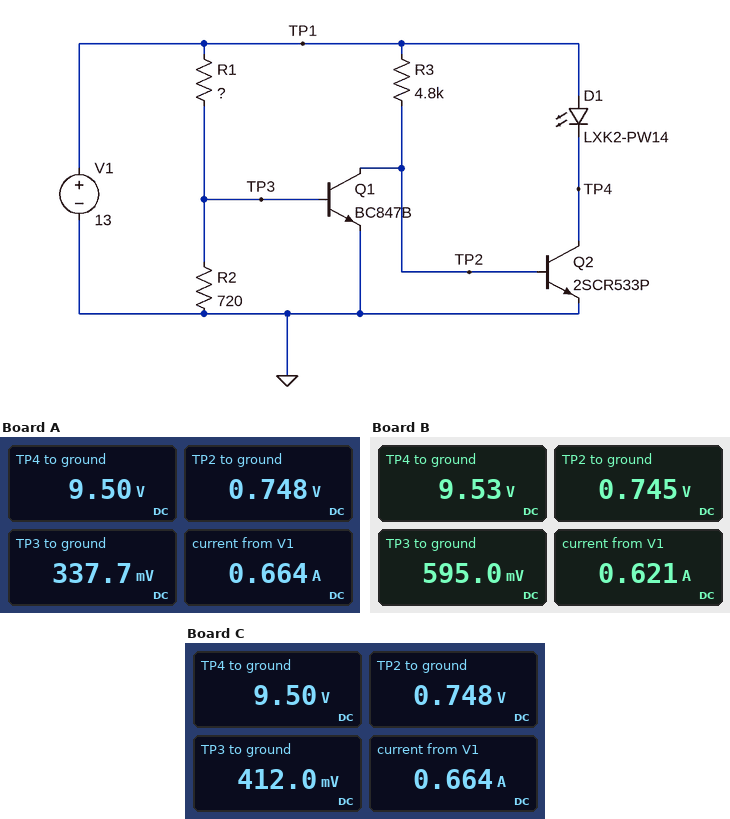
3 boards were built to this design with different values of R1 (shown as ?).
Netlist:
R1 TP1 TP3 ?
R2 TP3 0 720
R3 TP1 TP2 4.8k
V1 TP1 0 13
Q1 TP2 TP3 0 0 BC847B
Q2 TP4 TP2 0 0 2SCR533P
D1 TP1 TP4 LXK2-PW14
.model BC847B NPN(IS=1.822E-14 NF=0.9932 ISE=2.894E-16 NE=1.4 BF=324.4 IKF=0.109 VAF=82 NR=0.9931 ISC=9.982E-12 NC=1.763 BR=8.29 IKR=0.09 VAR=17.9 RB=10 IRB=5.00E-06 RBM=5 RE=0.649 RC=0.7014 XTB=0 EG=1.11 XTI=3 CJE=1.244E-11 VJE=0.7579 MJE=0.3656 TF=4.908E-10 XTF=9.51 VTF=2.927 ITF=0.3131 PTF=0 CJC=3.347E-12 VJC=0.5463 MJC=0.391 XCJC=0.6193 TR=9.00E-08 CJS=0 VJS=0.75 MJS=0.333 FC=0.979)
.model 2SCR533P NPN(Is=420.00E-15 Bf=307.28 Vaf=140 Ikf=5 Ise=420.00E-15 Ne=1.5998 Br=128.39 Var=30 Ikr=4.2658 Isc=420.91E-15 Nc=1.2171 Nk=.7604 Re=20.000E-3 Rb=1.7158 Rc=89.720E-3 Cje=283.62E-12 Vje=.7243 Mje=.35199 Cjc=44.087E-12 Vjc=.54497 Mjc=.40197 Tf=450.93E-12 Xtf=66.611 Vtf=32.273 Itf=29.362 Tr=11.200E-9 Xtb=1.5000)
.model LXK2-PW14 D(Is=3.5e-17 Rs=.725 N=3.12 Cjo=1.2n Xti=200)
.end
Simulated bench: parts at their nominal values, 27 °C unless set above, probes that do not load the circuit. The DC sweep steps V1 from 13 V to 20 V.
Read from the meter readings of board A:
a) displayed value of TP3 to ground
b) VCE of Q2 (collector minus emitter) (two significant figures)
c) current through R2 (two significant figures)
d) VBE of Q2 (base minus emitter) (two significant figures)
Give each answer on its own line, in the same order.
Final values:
337.7 mV
9.5 V
470 µA
750 mV
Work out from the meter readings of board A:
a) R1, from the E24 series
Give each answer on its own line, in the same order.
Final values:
27 kΩ
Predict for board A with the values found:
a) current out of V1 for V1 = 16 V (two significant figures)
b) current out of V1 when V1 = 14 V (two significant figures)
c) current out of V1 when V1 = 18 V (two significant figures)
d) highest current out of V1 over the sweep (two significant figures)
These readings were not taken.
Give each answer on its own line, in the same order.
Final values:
810 mA
710 mA
900 mA
990 mA
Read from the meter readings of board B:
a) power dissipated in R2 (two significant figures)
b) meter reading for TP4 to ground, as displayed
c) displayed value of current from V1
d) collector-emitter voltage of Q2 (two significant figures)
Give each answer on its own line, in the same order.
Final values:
490 µW
9.53 V
0.621 A
9.5 V
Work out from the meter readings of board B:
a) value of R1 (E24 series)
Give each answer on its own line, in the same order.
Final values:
15 kΩ
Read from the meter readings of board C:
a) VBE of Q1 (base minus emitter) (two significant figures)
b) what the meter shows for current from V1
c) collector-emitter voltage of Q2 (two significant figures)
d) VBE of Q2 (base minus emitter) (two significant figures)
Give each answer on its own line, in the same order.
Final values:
410 mV
0.664 A
9.5 V
750 mV
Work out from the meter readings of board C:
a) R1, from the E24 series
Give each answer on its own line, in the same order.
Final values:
22 kΩ
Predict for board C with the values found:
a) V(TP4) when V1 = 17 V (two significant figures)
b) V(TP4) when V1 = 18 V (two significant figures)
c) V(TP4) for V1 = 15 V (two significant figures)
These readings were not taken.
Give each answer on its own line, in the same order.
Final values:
13 V
14 V
11 V
